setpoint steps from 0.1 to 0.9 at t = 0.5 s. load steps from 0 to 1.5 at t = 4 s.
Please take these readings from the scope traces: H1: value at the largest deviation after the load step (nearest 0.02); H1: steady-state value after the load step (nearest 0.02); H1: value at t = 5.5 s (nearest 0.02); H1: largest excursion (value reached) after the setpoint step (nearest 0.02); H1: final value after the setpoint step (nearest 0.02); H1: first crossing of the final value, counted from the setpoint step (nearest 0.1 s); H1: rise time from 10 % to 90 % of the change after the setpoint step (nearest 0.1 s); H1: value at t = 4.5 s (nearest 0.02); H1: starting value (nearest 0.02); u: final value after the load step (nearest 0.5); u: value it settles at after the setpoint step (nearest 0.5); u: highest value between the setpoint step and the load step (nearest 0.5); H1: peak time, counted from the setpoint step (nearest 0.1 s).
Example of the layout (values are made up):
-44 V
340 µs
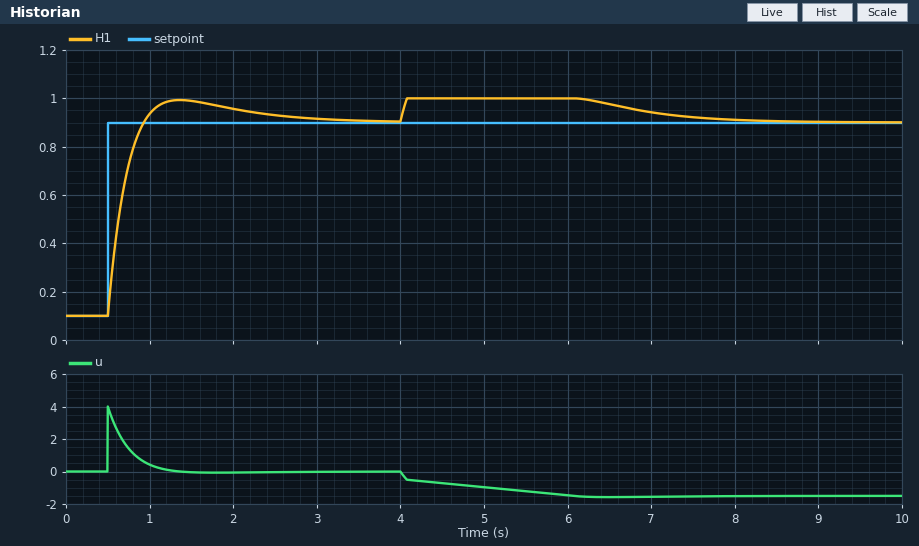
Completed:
1.00
0.90
1.00
1.00
0.90
0.4 s
0.3 s
1.00
0.10
-1.5
0.0
4.0
0.9 s
